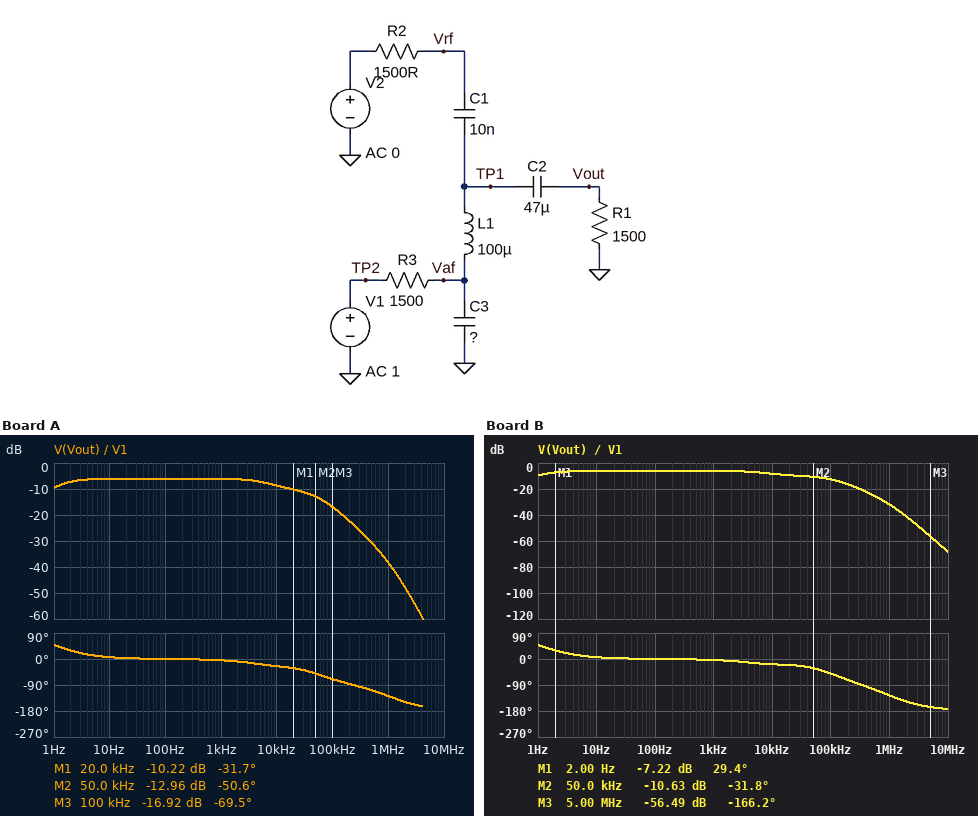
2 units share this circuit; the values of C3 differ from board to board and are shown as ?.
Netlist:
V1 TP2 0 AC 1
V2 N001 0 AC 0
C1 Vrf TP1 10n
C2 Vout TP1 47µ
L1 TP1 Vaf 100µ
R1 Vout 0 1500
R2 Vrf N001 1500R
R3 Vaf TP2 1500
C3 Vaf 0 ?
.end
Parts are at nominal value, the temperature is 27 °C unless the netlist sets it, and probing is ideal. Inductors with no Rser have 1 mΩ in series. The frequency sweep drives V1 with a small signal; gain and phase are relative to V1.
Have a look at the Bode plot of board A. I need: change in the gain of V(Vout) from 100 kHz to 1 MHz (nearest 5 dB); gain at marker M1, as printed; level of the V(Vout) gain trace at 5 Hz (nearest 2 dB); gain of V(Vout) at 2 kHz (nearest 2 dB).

-20 dB
-10.22 dB
-6 dB
-6 dB
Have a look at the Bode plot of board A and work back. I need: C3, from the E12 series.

6.8 nF
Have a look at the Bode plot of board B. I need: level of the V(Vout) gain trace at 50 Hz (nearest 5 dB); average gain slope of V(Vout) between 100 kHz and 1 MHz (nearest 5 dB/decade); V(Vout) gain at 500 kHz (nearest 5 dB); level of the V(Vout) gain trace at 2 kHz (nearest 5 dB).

-5 dB
-20 dB/decade
-25 dB
-5 dB
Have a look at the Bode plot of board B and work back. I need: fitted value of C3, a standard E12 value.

3.3 nF
